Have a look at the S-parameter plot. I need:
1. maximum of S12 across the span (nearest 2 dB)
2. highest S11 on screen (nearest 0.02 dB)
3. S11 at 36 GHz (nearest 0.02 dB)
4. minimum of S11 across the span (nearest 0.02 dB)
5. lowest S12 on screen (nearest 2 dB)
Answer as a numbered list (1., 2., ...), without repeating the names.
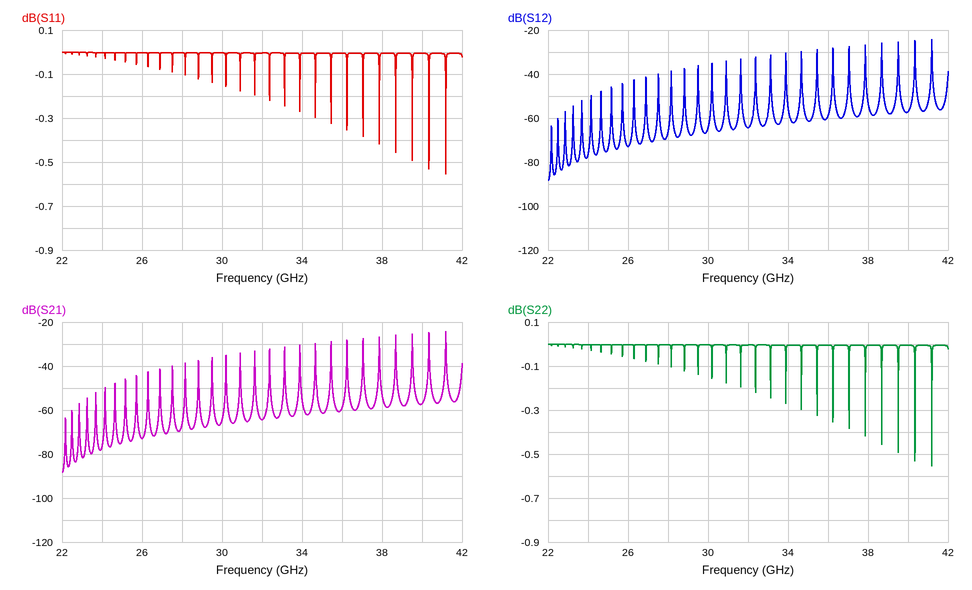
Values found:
1. -24 dB
2. 0.00 dB
3. 0.00 dB
4. -0.56 dB
5. -88 dB
